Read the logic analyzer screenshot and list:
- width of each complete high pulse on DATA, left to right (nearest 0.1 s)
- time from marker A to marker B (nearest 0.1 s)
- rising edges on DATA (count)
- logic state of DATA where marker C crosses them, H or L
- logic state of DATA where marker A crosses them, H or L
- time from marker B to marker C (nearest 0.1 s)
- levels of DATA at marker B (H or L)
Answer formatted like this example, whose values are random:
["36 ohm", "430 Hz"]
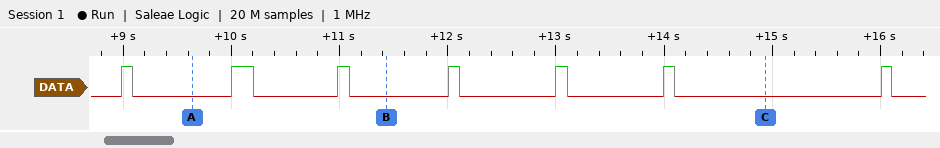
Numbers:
["0.1 s, 0.2 s, 0.1 s, 0.1 s, 0.1 s, 0.1 s, 0.1 s", "1.8 s", "7", "DATA=L", "DATA=L", "3.5 s", "DATA=L"]
